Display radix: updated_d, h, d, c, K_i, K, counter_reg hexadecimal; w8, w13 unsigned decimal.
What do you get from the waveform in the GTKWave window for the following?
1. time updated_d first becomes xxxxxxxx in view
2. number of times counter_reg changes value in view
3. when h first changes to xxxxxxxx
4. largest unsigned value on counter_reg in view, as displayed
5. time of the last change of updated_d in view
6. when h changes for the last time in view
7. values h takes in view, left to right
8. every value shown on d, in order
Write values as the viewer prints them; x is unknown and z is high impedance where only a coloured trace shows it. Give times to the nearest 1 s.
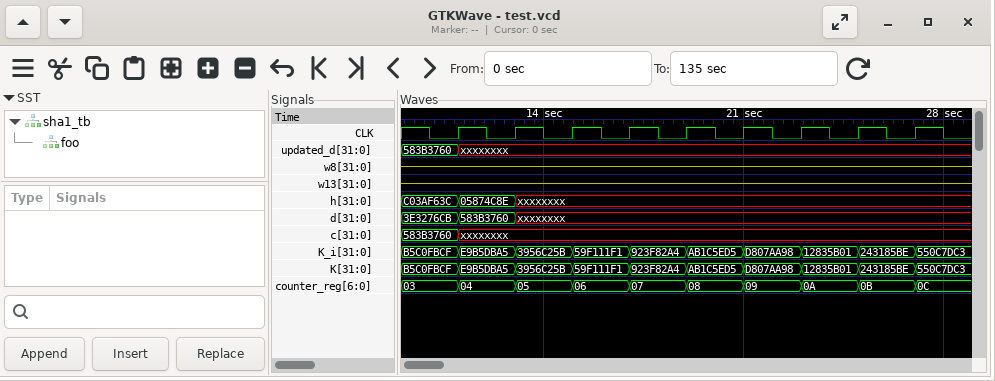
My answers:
11 s
9
13 s
0C
11 s
13 s
C03AF63C, 05874C8E, xxxxxxxx
3E3276CB, 583B3760, xxxxxxxx
